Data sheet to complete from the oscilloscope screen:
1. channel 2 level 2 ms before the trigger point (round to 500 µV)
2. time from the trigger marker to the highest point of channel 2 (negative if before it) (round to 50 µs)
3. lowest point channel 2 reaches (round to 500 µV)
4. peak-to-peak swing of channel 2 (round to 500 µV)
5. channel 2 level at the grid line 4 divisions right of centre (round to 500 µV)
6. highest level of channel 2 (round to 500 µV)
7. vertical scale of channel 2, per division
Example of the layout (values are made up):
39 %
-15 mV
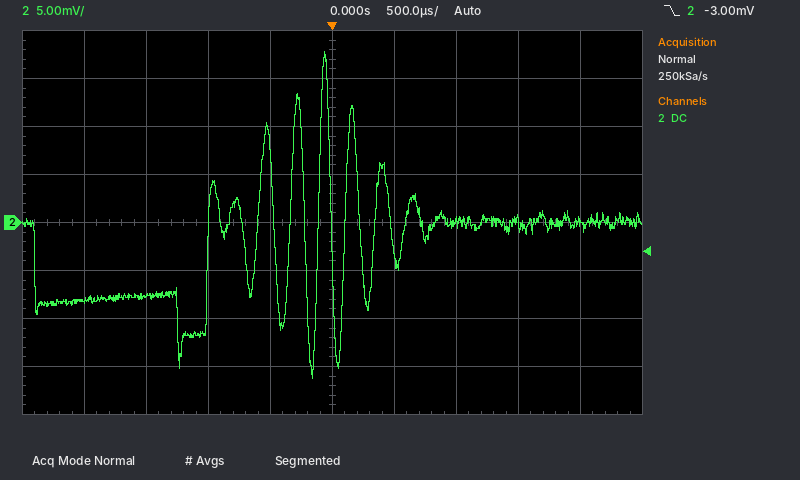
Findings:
-8.0 mV
-50 µs
-16.0 mV
34.0 mV
0.0 mV
18.0 mV
5 mV
